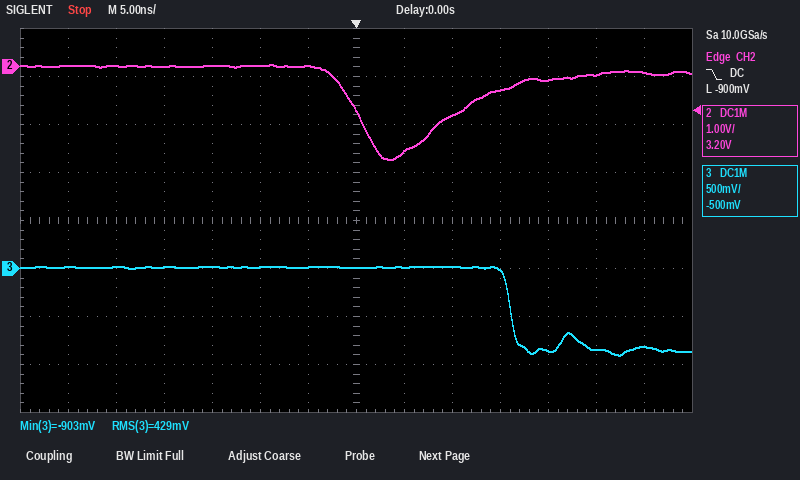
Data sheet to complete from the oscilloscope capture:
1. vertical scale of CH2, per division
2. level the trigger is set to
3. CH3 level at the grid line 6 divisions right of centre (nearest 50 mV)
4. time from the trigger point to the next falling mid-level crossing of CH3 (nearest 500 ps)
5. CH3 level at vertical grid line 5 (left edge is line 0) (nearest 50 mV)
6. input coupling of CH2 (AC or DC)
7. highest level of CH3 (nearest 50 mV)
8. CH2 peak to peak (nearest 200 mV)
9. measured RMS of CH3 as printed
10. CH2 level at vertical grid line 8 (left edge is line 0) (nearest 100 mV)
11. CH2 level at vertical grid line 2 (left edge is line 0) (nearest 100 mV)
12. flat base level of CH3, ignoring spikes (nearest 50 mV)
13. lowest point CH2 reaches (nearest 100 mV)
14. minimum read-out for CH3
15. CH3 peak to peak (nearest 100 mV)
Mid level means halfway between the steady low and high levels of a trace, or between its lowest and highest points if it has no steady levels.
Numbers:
1 V
-900 mV
-800 mV
16.0 ns
0 mV
DC
0 mV
2.0 V
429 mV
-1.8 V
0.0 V
-850 mV
-1.9 V
-903 mV
900 mV
